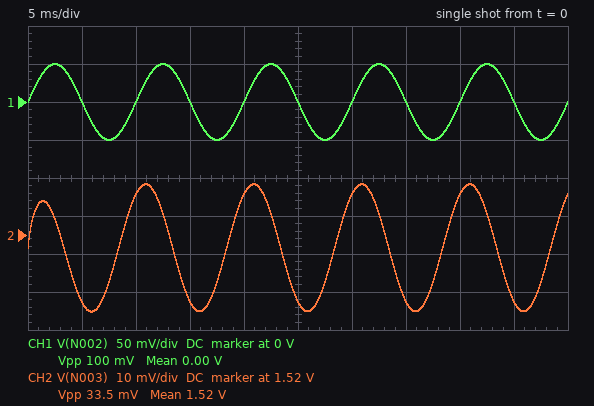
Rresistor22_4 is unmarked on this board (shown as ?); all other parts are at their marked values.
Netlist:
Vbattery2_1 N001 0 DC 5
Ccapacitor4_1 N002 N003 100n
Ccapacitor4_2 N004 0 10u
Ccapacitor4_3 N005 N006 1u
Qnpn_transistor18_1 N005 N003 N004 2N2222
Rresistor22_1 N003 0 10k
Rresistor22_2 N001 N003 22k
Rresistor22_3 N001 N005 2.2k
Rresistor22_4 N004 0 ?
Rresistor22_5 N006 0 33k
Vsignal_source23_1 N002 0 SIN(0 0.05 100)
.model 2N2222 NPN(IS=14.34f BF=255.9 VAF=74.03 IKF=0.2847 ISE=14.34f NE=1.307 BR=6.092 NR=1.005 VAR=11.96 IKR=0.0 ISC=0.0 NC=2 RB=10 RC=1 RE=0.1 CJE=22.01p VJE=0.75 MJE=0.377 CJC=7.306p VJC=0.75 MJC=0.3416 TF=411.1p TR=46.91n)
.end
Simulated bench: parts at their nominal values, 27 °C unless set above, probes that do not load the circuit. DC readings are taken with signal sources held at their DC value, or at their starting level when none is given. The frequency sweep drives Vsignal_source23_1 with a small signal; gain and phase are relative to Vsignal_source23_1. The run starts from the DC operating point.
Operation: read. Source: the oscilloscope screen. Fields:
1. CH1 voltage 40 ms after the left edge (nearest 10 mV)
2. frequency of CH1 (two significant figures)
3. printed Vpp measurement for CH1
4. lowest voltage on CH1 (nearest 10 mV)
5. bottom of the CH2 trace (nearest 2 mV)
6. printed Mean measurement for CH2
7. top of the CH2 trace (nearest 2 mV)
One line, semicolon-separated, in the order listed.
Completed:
0 V; 100 Hz; 100 mV; -50 mV; 1.500 V; 1.52 V; 1.534 V
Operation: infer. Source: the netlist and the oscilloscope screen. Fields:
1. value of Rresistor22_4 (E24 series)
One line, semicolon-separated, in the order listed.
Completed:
910 Ω
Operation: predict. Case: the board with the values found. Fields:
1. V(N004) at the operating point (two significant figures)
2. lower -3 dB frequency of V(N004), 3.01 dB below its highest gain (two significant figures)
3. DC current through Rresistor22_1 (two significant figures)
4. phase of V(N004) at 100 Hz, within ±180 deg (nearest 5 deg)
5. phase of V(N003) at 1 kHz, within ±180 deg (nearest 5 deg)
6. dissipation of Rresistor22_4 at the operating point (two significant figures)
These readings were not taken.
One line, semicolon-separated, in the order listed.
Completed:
870 mV; 110 Hz; 150 µA; 50 deg; 25 deg; 830 µW
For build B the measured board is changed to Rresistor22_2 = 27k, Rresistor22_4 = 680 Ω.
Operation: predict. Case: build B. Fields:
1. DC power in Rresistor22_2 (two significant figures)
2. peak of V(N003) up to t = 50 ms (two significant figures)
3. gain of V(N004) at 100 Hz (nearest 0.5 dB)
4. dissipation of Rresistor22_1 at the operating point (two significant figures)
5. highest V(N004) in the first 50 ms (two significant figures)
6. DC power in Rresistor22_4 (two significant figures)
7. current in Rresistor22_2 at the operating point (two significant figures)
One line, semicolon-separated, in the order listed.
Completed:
510 µW; 1.3 V; -9.5 dB; 170 µW; 670 mV; 630 µW; 140 µA
